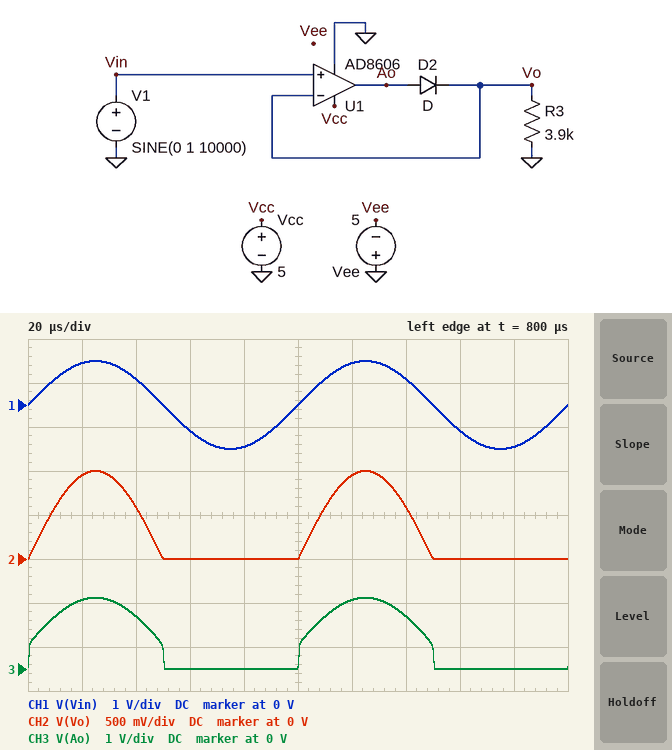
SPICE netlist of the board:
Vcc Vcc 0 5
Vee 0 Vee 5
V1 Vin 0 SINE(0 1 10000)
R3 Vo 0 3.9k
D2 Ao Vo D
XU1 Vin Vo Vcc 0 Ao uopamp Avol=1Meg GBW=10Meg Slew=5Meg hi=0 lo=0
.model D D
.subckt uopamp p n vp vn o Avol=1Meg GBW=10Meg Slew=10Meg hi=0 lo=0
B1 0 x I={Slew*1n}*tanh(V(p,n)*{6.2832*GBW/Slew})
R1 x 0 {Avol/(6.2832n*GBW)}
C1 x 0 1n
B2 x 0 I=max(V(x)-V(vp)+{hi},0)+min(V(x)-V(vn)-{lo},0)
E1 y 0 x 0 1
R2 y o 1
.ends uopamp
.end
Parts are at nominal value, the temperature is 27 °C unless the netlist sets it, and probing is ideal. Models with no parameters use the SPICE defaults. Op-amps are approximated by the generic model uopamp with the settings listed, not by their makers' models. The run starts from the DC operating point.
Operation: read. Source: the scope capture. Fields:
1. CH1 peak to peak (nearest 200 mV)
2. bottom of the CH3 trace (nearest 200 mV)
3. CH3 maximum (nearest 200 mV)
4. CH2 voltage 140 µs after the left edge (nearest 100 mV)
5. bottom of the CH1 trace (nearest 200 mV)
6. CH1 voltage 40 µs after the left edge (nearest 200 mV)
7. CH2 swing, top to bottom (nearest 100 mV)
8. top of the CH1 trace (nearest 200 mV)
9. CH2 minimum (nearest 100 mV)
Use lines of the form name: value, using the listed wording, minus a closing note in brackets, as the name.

CH1 peak to peak: 2.0 V
bottom of the CH3 trace: 0 V
CH3 maximum: 1.6 V
CH2 voltage 140 µs after the left edge: 600 mV
bottom of the CH1 trace: -1.0 V
CH1 voltage 40 µs after the left edge: 600 mV
CH2 swing, top to bottom: 1.0 V
top of the CH1 trace: 1.0 V
CH2 minimum: 0 V
